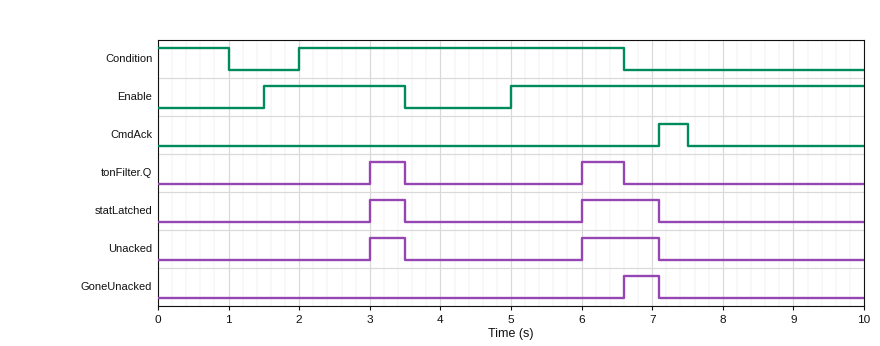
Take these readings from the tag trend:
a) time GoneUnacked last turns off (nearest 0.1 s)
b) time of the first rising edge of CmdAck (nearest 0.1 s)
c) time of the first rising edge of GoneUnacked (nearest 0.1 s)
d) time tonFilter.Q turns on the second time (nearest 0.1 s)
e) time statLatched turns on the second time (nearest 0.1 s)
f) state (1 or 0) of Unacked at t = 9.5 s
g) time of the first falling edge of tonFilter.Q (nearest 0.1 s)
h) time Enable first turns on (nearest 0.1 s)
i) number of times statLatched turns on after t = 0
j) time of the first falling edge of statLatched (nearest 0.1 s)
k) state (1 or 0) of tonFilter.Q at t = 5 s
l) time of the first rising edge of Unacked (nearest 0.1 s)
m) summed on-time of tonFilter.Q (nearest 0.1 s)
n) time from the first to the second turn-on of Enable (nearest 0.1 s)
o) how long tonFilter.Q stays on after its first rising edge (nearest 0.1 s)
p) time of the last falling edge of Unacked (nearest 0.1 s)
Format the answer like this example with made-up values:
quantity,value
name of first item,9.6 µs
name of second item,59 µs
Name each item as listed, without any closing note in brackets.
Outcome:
quantity,value
time GoneUnacked last turns off,7.1 s
time of the first rising edge of CmdAck,7.1 s
time of the first rising edge of GoneUnacked,6.6 s
time tonFilter.Q turns on the second time,6.0 s
time statLatched turns on the second time,6.0 s
state (1 or 0) of Unacked at t = 9.5 s,0
time of the first falling edge of tonFilter.Q,3.5 s
time Enable first turns on,1.5 s
number of times statLatched turns on after t = 0,2
time of the first falling edge of statLatched,3.5 s
state (1 or 0) of tonFilter.Q at t = 5 s,0
time of the first rising edge of Unacked,3.0 s
summed on-time of tonFilter.Q,1.1 s
time from the first to the second turn-on of Enable,3.5 s
how long tonFilter.Q stays on after its first rising edge,0.5 s
time of the last falling edge of Unacked,7.1 s
